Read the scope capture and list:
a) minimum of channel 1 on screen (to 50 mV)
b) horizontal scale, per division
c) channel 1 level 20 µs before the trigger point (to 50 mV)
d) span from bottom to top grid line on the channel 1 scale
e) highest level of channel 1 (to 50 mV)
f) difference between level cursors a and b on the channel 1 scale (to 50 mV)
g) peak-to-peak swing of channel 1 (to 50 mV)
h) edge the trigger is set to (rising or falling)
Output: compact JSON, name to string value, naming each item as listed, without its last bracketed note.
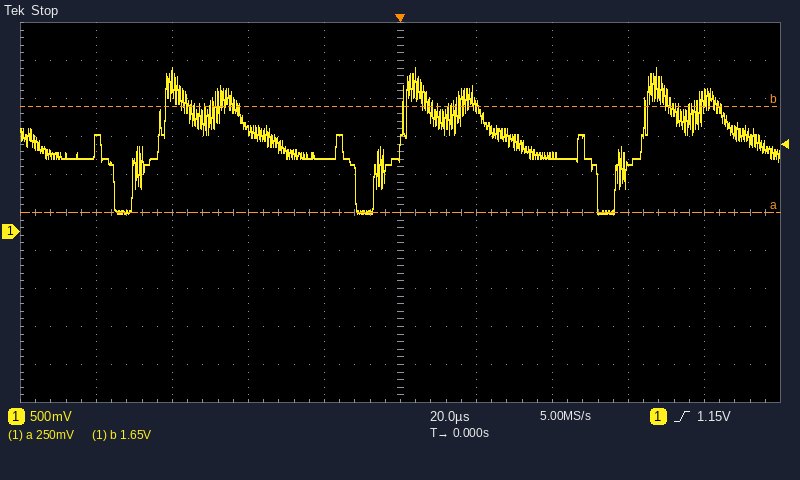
{"minimum of channel 1 on screen": "250 mV", "horizontal scale, per division": "20 µs", "channel 1 level 20 µs before the trigger point": "950 mV", "span from bottom to top grid line on the channel 1 scale": "5 V", "highest level of channel 1": "2.15 V", "difference between level cursors a and b on the channel 1 scale": "1.40 V", "peak-to-peak swing of channel 1": "1.90 V", "edge the trigger is set to": "rising"}
